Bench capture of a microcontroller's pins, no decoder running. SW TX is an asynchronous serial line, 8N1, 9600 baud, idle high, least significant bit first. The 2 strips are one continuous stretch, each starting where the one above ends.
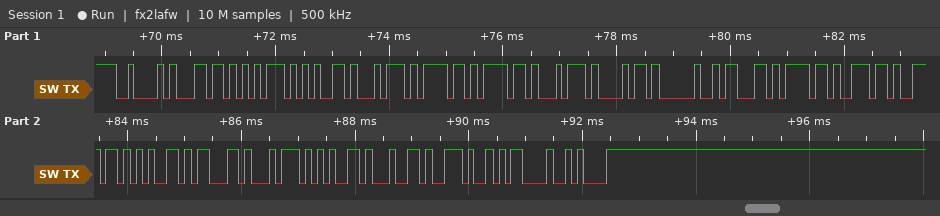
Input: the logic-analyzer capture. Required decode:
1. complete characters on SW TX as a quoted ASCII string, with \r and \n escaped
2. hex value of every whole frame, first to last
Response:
"Bluetooth connected.\r\n"
42 6C 75 65 74 6F 6F 74 68 20 63 6F 6E 6E 65 63 74 65 64 2E 0D 0A
